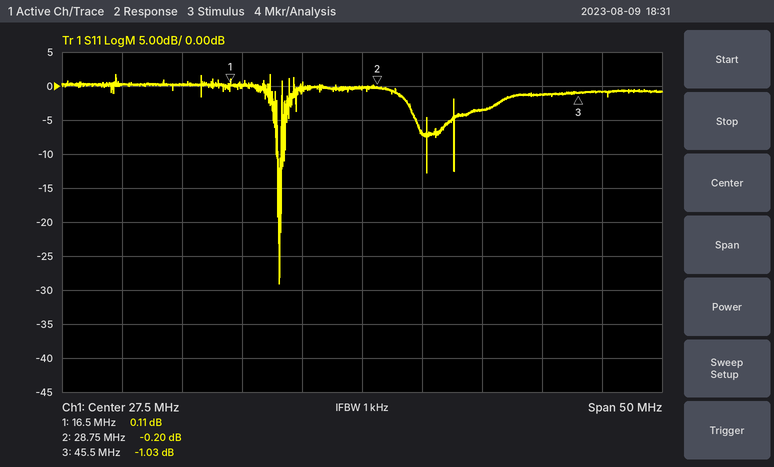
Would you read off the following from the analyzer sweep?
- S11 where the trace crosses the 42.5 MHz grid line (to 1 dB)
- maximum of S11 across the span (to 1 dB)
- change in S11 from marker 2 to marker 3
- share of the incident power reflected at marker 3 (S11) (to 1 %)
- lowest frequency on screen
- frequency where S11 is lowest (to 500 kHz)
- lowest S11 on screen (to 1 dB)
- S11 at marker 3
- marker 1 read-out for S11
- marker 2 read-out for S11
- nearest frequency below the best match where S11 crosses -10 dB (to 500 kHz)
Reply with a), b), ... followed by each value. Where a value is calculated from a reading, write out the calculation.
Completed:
a) -1 dB
b) 2 dB
c) -1.03 − (-0.2) = -0.83 dB
d) 10^(-1.03/10) ≈ 79 %
e) 2.5 MHz
f) 20.5 MHz
g) -29 dB
h) -1.03 dB
i) 0.11 dB
j) -0.20 dB
k) 20.5 MHz
